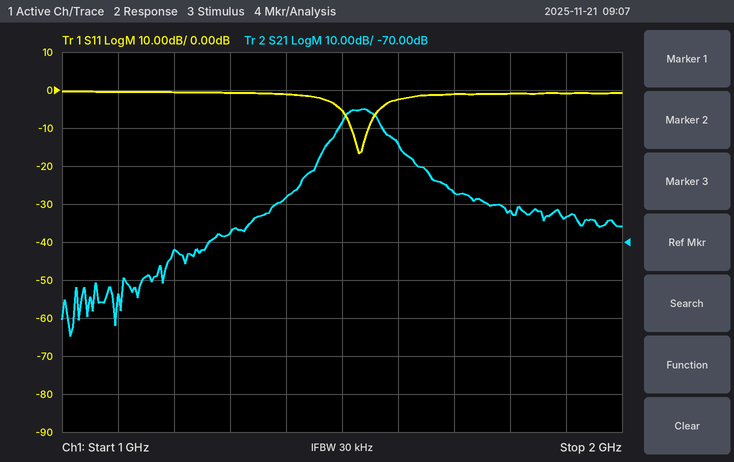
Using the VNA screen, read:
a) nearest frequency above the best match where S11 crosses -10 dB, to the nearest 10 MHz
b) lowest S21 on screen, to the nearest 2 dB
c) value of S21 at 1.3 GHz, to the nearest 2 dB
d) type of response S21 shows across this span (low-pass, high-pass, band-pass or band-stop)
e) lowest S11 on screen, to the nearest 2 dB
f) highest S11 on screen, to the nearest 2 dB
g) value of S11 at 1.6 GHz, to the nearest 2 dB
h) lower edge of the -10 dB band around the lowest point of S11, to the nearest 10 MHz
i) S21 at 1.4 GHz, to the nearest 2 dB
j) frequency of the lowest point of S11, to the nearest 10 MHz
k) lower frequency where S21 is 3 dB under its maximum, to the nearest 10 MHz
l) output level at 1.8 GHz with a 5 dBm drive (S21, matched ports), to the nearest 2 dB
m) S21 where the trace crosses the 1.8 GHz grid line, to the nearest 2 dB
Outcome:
1.55 GHz
-94 dB
-68 dB
band-pass
-16 dB
0 dB
-2 dB
1.52 GHz
-58 dB
1.53 GHz
1.50 GHz
-56 dBm
-62 dB
